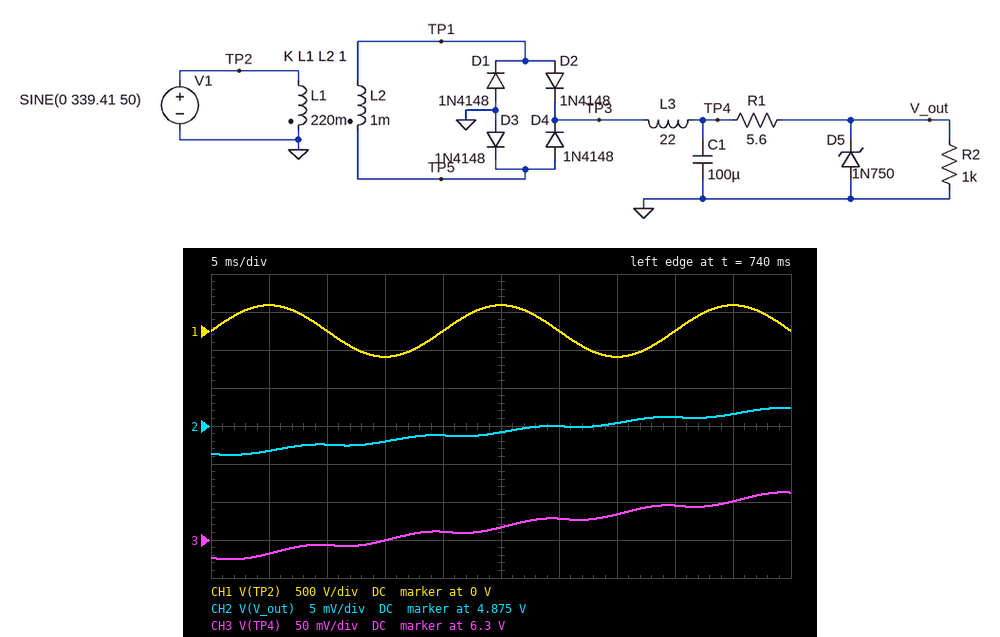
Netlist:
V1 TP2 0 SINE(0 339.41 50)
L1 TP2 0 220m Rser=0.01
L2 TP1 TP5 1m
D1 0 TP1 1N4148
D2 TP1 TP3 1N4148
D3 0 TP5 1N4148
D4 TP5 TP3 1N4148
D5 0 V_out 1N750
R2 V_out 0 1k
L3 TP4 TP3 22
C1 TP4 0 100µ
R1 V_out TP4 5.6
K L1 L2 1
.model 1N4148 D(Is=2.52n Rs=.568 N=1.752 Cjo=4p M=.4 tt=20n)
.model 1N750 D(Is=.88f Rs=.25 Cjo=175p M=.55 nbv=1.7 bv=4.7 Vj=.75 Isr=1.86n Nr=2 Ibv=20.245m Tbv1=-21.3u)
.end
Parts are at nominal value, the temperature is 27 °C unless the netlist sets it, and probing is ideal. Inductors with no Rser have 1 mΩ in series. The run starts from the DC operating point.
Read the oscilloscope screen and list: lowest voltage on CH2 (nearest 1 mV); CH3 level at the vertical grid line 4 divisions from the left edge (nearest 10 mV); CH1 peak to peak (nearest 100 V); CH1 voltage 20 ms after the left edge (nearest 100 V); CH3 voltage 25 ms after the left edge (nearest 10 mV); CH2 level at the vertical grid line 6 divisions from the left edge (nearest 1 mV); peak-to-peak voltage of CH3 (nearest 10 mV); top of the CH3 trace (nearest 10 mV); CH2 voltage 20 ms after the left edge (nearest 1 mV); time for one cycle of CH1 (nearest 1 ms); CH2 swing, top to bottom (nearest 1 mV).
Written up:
4.871 V
6.31 V
700 V
0 V
6.32 V
4.875 V
90 mV
6.36 V
4.874 V
20 ms
6 mV
